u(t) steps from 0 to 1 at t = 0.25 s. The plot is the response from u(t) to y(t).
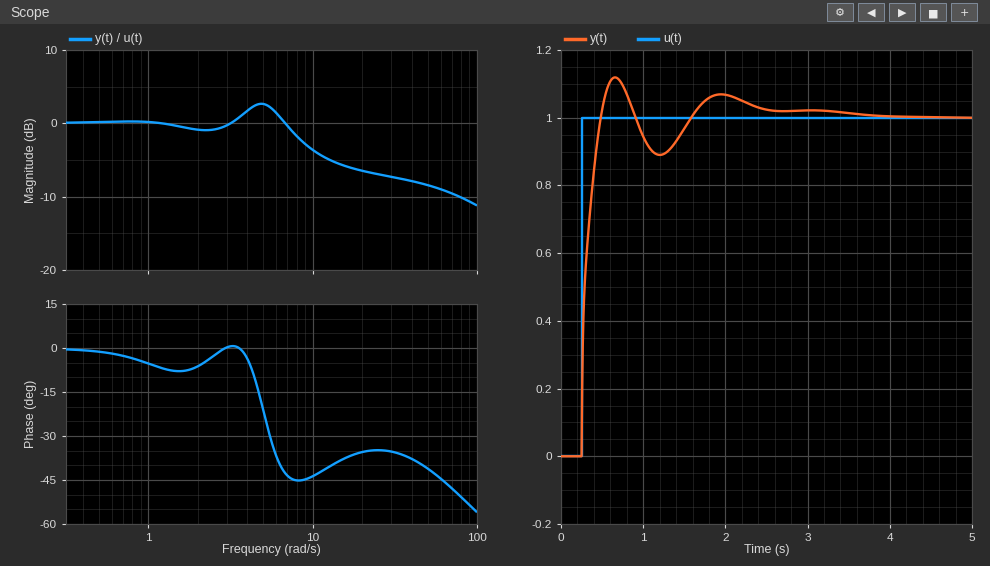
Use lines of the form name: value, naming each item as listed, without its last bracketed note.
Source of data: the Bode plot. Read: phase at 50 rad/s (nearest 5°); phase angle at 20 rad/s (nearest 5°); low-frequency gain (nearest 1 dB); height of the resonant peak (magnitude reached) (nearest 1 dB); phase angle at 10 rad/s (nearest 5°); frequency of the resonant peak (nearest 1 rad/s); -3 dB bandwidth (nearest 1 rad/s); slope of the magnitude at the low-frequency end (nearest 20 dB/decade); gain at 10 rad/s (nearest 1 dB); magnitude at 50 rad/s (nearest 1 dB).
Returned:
phase at 50 rad/s: -40°
phase angle at 20 rad/s: -35°
low-frequency gain: 0 dB
height of the resonant peak (magnitude reached): 3 dB
phase angle at 10 rad/s: -45°
frequency of the resonant peak: 5 rad/s
-3 dB bandwidth: 9 rad/s
slope of the magnitude at the low-frequency end: 0 dB/decade
gain at 10 rad/s: -4 dB
magnitude at 50 rad/s: -8 dB
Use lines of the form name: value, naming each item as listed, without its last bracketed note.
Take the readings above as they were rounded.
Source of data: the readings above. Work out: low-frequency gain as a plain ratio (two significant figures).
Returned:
low-frequency gain as a plain ratio: 1.0
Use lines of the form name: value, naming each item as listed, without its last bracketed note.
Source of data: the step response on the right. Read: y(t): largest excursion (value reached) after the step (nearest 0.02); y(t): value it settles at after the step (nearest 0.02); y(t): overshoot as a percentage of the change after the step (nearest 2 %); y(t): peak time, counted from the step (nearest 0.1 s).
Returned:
y(t): largest excursion (value reached) after the step: 1.12
y(t): value it settles at after the step: 1.00
y(t): overshoot as a percentage of the change after the step: 12 %
y(t): peak time, counted from the step: 0.4 s
